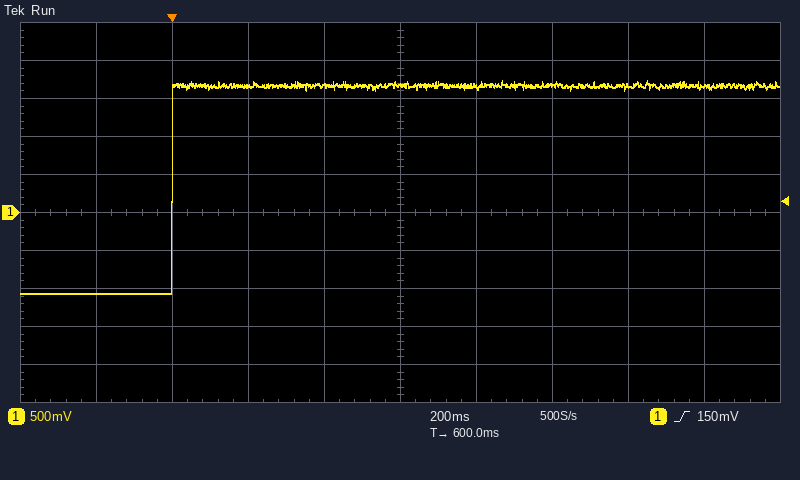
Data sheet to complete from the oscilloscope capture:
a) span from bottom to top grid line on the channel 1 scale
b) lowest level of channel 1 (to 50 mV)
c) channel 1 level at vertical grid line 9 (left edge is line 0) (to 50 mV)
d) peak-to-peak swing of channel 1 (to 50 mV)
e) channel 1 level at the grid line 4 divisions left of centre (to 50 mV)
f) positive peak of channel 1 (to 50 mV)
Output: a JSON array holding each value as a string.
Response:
["5 V", "-1.05 V", "1.65 V", "2.80 V", "-1.05 V", "1.75 V"]
